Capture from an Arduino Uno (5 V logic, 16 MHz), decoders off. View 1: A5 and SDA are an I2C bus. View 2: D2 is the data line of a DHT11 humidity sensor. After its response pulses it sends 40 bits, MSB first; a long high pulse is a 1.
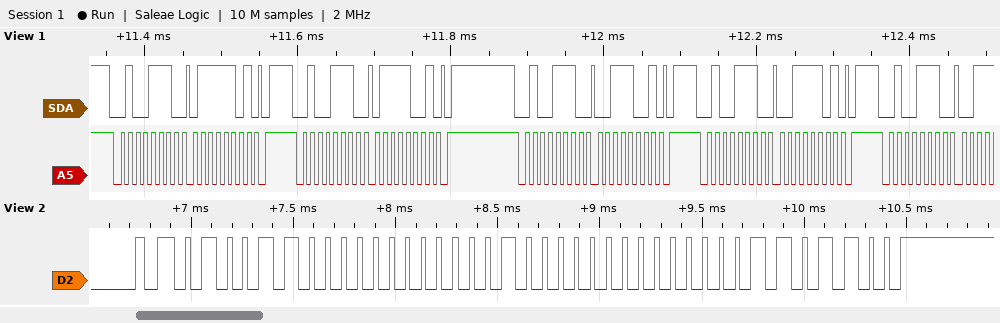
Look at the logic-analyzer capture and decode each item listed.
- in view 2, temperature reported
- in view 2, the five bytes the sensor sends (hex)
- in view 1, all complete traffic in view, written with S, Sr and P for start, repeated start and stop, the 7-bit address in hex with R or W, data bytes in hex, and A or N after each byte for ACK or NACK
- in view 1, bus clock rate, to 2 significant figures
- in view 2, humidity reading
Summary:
32.0 °C
4C 00 20 00 6C
S 27W A 7D A P S 27W A 79 A P S 27W A 39 A P S 27W A 3D A P S 27W A
100 kHz
76 %
